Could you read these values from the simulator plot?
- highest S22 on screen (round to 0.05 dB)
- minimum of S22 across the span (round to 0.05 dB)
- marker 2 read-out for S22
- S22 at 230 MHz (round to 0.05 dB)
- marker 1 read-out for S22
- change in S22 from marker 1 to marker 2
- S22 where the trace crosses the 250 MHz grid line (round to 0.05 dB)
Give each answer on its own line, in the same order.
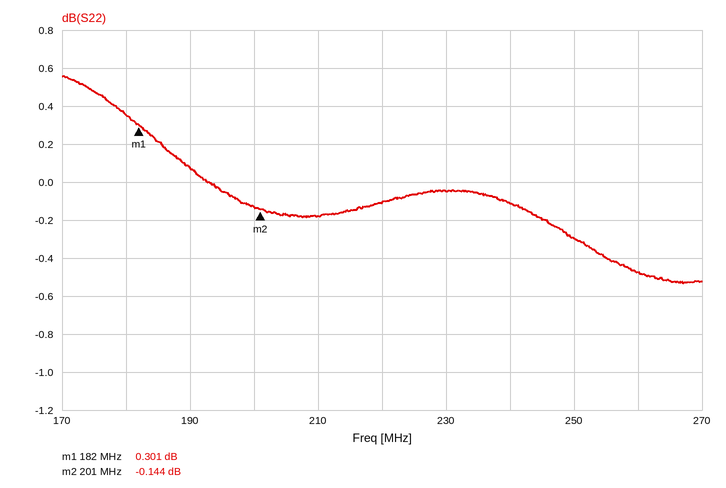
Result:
0.55 dB
-0.55 dB
-0.144 dB
-0.05 dB
0.301 dB
-0.445 dB
-0.30 dB
